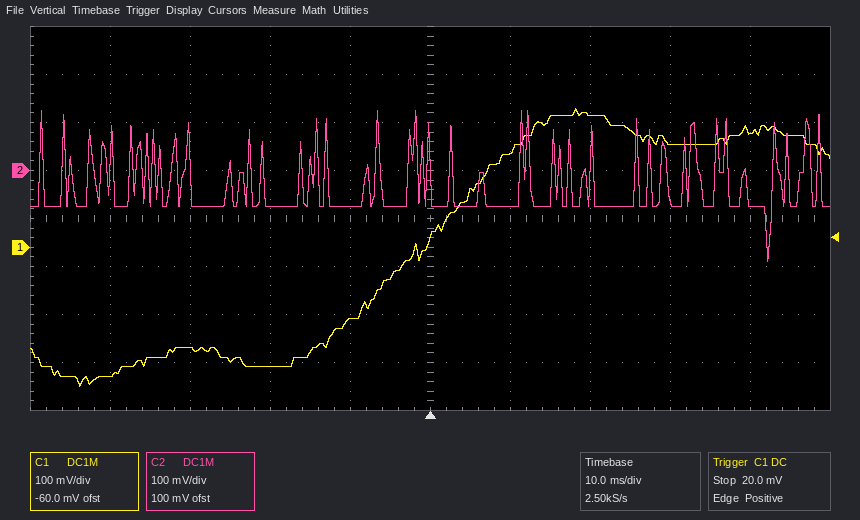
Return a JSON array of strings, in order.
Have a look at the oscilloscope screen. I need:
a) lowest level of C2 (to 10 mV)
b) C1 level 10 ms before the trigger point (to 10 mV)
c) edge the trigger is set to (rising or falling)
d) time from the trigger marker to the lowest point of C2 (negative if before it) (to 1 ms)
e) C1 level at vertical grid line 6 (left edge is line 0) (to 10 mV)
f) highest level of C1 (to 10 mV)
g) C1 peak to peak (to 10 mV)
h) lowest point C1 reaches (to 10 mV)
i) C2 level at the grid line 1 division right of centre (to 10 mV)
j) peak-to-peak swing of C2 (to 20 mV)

["-190 mV", "-150 mV", "rising", "+42 ms", "200 mV", "290 mV", "580 mV", "-290 mV", "-80 mV", "320 mV"]
